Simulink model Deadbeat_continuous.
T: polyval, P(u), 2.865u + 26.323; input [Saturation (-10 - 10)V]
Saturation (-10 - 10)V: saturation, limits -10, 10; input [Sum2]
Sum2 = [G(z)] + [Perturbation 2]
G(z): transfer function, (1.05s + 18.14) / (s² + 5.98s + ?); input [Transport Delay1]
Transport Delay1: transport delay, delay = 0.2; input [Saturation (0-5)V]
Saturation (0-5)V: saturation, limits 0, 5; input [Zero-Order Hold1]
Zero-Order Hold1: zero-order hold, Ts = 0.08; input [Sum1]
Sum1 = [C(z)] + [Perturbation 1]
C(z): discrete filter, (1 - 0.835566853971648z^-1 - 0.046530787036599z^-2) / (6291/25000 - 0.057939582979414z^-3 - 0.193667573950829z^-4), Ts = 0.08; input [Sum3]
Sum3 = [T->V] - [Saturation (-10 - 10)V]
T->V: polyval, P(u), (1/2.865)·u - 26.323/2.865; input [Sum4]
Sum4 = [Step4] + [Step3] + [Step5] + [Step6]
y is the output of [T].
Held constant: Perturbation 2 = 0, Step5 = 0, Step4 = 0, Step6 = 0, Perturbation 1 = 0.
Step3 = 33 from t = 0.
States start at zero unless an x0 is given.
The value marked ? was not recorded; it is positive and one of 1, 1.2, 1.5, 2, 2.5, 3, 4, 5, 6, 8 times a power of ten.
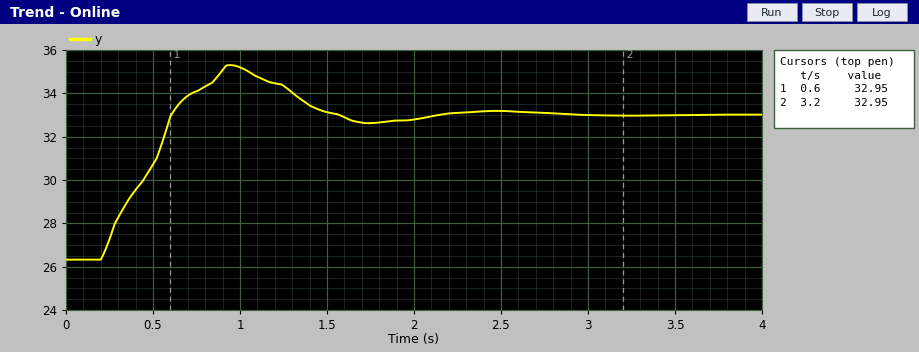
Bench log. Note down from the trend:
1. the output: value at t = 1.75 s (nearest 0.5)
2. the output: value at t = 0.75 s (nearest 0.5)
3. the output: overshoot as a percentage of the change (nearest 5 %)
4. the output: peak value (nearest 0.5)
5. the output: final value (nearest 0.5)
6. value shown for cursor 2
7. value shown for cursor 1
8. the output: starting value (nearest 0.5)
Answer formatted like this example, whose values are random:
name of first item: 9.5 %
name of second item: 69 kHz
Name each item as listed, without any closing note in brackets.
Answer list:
the output: value at t = 1.75 s: 32.5
the output: value at t = 0.75 s: 34.0
the output: overshoot as a percentage of the change: 35 %
the output: peak value: 35.5
the output: final value: 33.0
value shown for cursor 2: 32.95
value shown for cursor 1: 32.95
the output: starting value: 26.5
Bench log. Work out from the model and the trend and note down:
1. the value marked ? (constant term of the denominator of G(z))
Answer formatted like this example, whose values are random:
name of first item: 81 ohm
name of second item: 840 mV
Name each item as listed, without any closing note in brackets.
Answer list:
the value marked ? (constant term of the denominator of G(z)): 8
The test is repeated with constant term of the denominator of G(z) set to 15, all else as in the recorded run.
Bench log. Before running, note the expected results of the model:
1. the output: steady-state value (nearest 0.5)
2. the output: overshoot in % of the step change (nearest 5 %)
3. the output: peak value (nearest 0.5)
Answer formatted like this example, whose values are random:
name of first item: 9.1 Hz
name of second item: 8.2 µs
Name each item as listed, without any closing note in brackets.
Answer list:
the output: steady-state value: 33.0
the output: overshoot in % of the step change: 10 %
the output: peak value: 33.5
